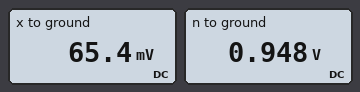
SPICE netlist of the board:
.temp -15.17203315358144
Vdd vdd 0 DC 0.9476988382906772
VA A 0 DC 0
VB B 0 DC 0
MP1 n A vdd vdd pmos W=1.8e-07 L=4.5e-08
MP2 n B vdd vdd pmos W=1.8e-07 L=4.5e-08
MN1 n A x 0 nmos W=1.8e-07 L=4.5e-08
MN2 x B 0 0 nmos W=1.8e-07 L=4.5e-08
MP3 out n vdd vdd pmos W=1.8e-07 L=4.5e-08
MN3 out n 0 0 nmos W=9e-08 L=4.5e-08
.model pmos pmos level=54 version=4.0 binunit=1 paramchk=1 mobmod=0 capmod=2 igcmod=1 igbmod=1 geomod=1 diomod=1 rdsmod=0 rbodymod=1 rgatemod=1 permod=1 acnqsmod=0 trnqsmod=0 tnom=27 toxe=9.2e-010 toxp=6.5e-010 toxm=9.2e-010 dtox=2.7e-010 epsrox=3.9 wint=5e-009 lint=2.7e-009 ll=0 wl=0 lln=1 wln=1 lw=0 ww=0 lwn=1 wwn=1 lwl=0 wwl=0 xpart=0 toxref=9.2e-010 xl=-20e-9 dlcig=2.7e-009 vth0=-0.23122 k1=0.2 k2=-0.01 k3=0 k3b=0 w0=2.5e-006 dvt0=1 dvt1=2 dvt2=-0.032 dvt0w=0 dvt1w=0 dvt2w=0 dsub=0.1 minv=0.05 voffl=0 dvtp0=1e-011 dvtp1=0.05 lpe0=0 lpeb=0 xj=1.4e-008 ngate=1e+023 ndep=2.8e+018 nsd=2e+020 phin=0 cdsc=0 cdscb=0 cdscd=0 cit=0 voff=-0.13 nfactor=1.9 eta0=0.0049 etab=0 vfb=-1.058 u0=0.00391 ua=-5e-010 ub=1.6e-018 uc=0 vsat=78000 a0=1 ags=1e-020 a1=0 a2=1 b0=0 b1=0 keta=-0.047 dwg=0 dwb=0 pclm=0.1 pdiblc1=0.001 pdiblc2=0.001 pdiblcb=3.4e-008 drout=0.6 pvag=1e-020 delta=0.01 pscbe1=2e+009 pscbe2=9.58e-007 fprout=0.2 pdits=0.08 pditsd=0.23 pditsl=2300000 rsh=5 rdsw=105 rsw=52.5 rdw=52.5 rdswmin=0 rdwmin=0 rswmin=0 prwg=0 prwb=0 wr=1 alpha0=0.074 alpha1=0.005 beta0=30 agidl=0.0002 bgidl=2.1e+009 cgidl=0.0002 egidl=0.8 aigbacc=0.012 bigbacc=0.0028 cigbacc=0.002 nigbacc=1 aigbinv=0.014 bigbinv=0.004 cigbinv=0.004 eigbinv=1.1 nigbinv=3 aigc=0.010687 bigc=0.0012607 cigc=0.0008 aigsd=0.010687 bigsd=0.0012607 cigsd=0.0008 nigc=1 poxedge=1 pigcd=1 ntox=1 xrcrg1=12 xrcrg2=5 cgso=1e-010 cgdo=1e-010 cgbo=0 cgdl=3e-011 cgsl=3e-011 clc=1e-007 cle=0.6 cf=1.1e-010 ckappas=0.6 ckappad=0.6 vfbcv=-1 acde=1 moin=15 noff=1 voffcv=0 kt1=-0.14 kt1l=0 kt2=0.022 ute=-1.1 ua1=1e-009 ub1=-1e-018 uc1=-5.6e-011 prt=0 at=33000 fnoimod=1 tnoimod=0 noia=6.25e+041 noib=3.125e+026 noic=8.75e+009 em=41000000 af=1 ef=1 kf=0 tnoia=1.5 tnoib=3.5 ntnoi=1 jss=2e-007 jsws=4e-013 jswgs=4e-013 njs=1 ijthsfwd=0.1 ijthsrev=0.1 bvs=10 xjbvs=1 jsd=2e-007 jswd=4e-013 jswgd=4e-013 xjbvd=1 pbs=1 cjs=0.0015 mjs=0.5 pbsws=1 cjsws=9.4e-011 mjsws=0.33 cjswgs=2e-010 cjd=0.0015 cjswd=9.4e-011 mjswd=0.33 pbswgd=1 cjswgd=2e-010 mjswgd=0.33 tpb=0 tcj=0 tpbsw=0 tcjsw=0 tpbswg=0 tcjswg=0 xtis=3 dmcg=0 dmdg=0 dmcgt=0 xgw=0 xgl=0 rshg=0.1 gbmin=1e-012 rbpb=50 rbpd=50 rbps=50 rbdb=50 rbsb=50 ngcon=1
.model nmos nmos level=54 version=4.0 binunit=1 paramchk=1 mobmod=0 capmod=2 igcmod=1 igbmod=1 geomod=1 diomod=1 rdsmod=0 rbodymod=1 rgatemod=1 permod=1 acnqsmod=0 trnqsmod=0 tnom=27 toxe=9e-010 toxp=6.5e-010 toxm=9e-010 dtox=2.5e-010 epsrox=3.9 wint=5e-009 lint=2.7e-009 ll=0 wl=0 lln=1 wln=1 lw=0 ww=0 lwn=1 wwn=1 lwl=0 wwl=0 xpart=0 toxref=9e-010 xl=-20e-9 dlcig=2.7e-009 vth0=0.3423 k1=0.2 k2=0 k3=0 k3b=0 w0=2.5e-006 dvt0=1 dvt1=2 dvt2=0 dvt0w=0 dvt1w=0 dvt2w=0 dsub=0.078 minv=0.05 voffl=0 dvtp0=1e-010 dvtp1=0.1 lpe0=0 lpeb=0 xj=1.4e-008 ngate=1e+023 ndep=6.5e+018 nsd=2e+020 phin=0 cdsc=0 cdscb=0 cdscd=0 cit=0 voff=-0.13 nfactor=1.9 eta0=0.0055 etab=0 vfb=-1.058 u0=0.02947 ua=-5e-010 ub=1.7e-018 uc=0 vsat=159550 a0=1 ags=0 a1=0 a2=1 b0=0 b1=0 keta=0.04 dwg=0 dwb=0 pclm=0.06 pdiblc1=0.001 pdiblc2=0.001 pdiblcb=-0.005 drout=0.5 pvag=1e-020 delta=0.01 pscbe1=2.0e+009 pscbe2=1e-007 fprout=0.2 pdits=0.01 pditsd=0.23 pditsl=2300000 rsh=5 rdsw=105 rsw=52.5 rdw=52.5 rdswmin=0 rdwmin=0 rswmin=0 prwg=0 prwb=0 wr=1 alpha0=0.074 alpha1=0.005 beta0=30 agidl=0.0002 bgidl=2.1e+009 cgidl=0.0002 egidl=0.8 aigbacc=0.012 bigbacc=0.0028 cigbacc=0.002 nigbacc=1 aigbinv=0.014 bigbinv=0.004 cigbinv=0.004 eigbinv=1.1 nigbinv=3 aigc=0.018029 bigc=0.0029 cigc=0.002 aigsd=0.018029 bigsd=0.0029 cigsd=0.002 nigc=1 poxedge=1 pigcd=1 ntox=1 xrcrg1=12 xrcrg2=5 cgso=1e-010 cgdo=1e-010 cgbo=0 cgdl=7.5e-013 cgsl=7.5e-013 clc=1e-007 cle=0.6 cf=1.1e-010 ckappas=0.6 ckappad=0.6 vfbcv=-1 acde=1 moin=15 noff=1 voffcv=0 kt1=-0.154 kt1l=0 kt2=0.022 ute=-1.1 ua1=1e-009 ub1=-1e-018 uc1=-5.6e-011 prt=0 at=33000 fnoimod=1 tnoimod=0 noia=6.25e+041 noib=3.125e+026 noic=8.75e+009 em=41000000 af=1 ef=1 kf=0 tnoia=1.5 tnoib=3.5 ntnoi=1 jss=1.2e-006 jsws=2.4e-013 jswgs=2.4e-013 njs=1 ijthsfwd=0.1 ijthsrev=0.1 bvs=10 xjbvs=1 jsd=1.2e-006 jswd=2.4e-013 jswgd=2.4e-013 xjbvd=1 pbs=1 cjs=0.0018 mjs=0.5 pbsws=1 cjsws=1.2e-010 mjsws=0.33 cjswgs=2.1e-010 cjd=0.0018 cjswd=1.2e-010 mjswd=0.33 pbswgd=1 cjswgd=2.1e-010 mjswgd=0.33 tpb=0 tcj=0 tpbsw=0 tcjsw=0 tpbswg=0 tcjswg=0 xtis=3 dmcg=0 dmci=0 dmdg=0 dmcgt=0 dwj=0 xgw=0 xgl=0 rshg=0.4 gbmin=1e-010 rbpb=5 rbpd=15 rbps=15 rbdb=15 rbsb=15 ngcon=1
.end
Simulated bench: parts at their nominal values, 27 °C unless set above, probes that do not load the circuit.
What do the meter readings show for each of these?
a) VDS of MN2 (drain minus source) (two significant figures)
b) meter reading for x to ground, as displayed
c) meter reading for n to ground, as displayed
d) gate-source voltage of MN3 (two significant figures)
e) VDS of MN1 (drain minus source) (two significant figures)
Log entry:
65 mV
65.4 mV
0.948 V
950 mV
880 mV
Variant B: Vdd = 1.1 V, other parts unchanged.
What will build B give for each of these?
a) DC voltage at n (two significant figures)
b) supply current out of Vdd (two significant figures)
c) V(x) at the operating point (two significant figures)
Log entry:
1.1 V
250 nA
75 mV
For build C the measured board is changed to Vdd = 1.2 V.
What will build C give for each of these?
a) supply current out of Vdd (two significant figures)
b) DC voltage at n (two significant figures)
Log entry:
390 nA
1.2 V
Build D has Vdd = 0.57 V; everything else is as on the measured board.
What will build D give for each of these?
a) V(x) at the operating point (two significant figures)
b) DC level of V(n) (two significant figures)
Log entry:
42 mV
570 mV
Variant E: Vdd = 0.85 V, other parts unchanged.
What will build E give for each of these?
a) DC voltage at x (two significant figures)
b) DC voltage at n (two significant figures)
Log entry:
59 mV
850 mV
